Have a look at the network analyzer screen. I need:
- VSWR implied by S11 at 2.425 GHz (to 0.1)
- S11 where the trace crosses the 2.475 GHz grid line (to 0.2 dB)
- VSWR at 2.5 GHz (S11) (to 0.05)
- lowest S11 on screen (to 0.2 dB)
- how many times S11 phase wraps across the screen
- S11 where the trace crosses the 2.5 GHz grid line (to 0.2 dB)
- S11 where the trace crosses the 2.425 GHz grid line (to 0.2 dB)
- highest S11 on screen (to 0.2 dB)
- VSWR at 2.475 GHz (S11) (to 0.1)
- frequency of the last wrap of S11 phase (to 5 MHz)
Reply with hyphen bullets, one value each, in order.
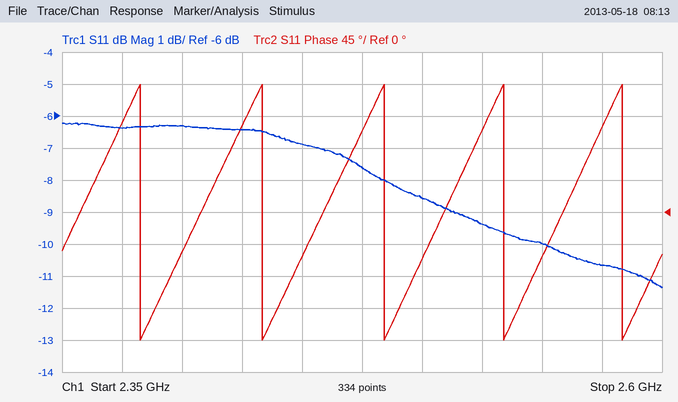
- 2.8
- -7.6 dB
- 2.20
- -11.4 dB
- 5
- -8.6 dB
- -6.4 dB
- -6.2 dB
- 2.4
- 2.585 GHz
